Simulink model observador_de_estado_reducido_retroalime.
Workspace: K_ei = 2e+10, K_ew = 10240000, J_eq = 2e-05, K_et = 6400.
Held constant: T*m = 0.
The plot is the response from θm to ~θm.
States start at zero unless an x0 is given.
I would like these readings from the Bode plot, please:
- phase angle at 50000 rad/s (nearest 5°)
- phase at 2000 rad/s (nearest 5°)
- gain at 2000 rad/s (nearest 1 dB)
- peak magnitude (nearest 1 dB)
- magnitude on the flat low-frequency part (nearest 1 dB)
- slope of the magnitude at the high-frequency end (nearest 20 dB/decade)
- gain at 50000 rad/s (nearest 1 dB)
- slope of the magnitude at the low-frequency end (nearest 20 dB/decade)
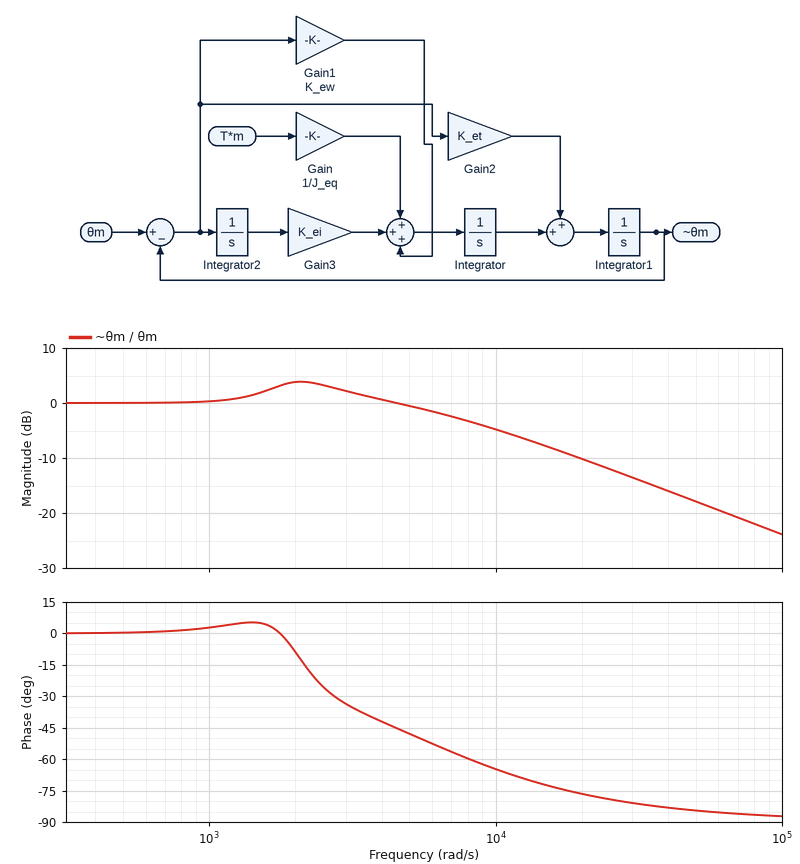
-85°
-10°
4 dB
4 dB
0 dB
-20 dB/decade
-18 dB
0 dB/decade
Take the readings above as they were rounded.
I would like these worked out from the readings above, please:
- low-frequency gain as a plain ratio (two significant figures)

1.0
